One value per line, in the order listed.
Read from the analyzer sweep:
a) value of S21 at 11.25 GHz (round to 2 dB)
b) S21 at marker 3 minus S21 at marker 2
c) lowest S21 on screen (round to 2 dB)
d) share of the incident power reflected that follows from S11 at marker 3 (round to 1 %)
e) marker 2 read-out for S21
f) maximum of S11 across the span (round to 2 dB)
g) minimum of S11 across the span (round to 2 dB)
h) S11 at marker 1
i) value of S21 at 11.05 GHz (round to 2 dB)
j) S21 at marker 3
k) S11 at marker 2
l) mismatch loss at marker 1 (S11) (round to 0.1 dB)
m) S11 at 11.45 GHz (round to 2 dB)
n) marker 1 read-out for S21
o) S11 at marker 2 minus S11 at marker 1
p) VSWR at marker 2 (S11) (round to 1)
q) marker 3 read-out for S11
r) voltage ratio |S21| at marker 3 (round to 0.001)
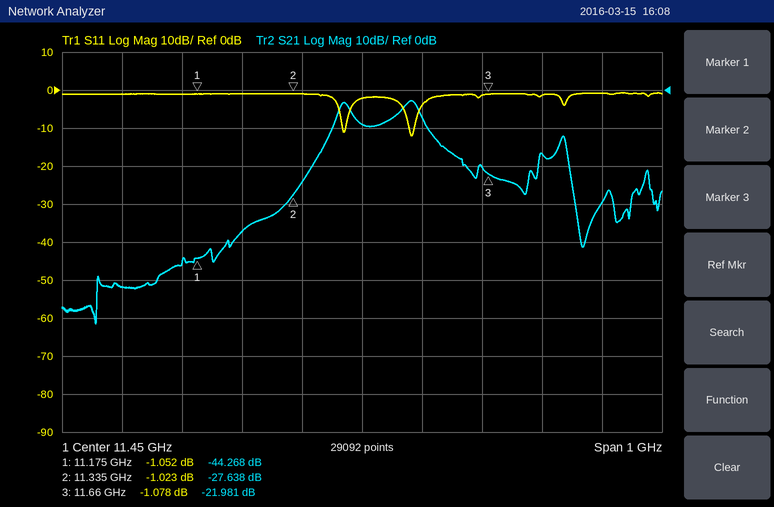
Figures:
-38 dB
5.657 dB
-62 dB
78 %
-27.638 dB
0 dB
-12 dB
-1.052 dB
-52 dB
-21.981 dB
-1.023 dB
6.7 dB
-2 dB
-44.268 dB
0.029 dB
17
-1.078 dB
0.080
